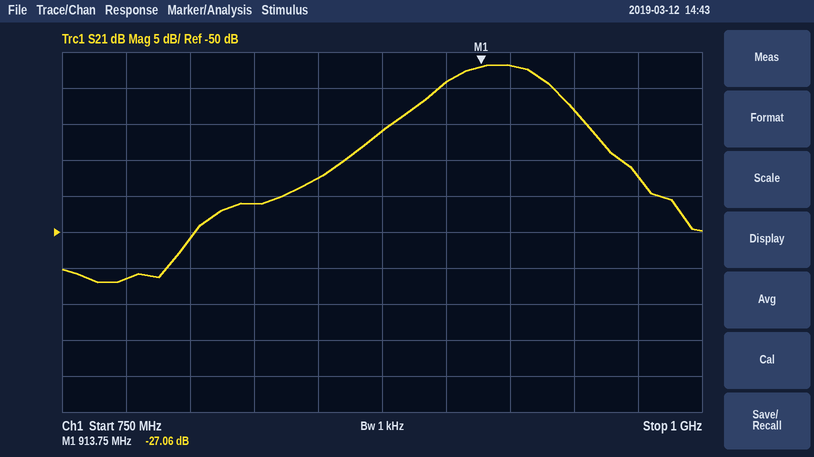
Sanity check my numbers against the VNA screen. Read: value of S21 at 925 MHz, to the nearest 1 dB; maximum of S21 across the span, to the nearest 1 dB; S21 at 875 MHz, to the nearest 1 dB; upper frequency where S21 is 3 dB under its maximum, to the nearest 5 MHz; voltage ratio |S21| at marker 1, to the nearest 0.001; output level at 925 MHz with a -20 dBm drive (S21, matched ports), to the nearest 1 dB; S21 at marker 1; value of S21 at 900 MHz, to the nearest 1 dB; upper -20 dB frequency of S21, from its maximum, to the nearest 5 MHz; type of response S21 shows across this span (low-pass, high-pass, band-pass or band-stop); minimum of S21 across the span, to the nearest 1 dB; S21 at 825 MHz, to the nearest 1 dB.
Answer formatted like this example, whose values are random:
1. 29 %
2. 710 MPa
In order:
1. -27 dB
2. -27 dB
3. -36 dB
4. 940 MHz
5. 0.044
6. -47 dBm
7. -27.06 dB
8. -29 dB
9. 990 MHz
10. band-pass
11. -57 dB
12. -46 dB
